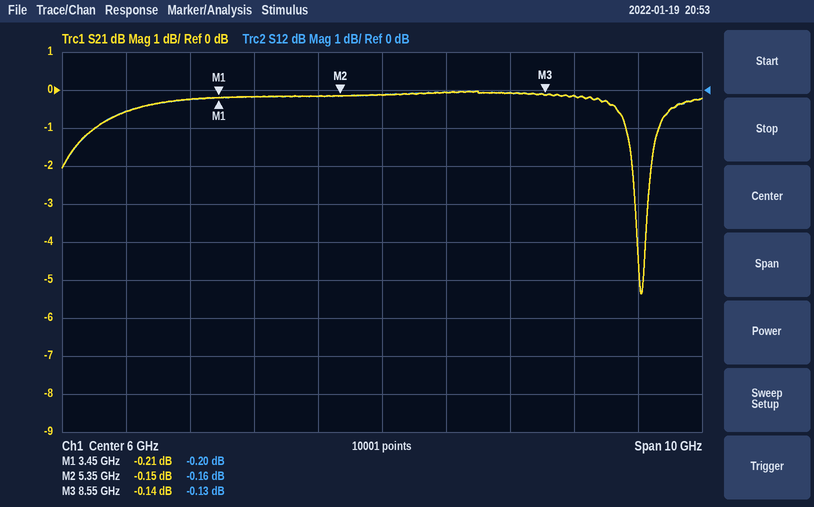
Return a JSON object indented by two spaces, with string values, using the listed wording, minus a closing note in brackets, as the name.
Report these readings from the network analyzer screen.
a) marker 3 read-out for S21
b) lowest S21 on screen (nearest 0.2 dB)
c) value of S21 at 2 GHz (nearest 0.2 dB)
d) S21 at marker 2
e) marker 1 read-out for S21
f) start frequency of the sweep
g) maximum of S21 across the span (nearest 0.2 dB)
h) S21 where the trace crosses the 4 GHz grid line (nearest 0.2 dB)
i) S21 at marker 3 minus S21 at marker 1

{
  "marker 3 read-out for S21": "-0.14 dB",
  "lowest S21 on screen": "-5.4 dB",
  "value of S21 at 2 GHz": "-0.6 dB",
  "S21 at marker 2": "-0.15 dB",
  "marker 1 read-out for S21": "-0.21 dB",
  "start frequency of the sweep": "1 GHz",
  "maximum of S21 across the span": "0.0 dB",
  "S21 where the trace crosses the 4 GHz grid line": "-0.2 dB",
  "S21 at marker 3 minus S21 at marker 1": "0.07 dB"
}
